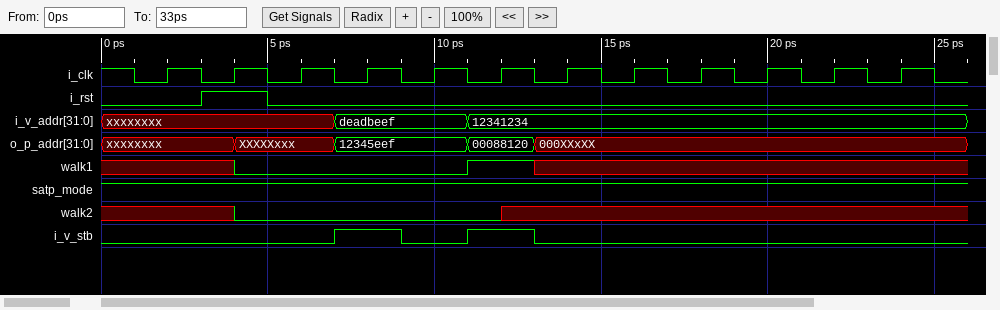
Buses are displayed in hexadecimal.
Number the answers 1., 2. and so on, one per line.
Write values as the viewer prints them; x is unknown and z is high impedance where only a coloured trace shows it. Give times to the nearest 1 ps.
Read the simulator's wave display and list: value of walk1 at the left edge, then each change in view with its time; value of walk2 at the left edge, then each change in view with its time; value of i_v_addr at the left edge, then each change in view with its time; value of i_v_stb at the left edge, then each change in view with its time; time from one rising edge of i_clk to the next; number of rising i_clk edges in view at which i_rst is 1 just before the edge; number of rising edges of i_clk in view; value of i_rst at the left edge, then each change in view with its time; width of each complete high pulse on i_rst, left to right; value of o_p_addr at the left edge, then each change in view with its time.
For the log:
1. x, 0 at 4 ps, 1 at 11 ps, x at 13 ps
2. x, 0 at 4 ps, x at 12 ps
3. xxxxxxxx, deadbeef at 7 ps, 12341234 at 11 ps
4. 0, 1 at 7 ps, 0 at 9 ps, 1 at 11 ps, 0 at 13 ps
5. 2 ps
6. 1
7. 12
8. 0, 1 at 3 ps, 0 at 5 ps
9. 2 ps
10. xxxxxxxx, XXXXXxxx at 4 ps, 12345eef at 7 ps, 00088120 at 11 ps, 000XXxXX at 13 ps
